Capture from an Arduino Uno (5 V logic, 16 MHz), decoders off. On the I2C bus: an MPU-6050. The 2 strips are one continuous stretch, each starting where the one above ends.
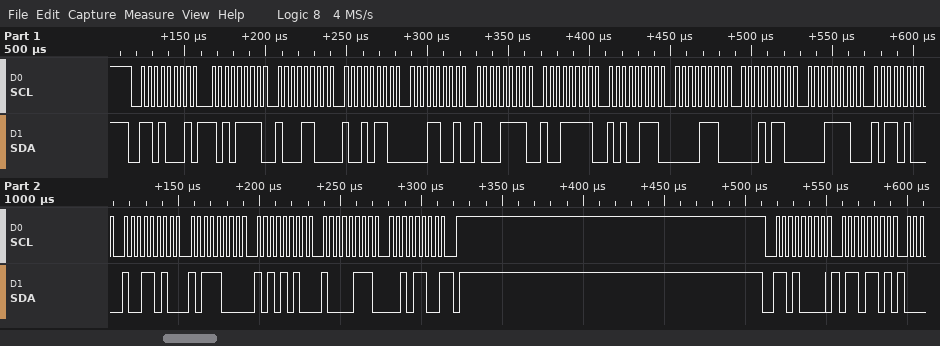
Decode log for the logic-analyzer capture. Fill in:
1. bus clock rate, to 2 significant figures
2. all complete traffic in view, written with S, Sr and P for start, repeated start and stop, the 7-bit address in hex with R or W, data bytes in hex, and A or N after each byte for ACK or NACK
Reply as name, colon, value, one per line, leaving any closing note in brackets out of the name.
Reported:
bus clock rate, to 2 significant figures: 250 kHz
all complete traffic in view, written with S, Sr and P for start, repeated start and stop, the 7-bit address in hex with R or W, data bytes in hex, and A or N after each byte for ACK or NACK: S 68R A AF A 8C A 96 A 19 A 8F A 9F A A7 A 0E A 16 A 1E A B4 A 9A A B8 A AA A 87 A 2C N P S 68W A 6D A
